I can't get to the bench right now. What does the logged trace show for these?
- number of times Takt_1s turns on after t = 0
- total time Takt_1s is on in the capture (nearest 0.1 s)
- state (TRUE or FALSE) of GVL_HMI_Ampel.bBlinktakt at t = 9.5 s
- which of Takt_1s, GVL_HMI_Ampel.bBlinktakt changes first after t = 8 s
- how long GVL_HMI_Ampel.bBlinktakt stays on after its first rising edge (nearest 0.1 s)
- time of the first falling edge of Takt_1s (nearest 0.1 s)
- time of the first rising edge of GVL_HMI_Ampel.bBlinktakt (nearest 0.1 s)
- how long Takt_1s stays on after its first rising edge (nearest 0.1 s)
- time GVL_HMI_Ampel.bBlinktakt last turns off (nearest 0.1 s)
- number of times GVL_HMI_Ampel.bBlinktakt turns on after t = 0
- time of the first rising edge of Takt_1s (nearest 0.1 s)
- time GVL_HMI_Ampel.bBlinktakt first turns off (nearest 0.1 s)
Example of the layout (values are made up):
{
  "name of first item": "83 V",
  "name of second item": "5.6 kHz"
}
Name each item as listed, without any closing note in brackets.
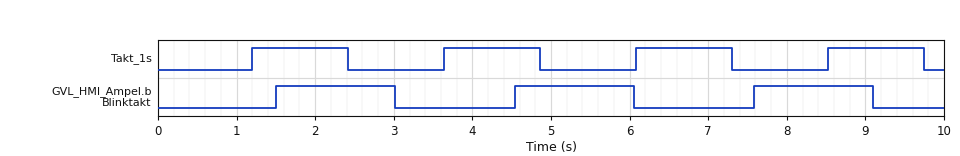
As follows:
{
  "number of times Takt_1s turns on after t = 0": "4",
  "total time Takt_1s is on in the capture": "4.9 s",
  "state (TRUE or FALSE) of GVL_HMI_Ampel.bBlinktakt at t = 9.5 s": "FALSE",
  "which of Takt_1s, GVL_HMI_Ampel.bBlinktakt changes first after t = 8 s": "Takt_1s",
  "how long GVL_HMI_Ampel.bBlinktakt stays on after its first rising edge": "1.5 s",
  "time of the first falling edge of Takt_1s": "2.4 s",
  "time of the first rising edge of GVL_HMI_Ampel.bBlinktakt": "1.5 s",
  "how long Takt_1s stays on after its first rising edge": "1.2 s",
  "time GVL_HMI_Ampel.bBlinktakt last turns off": "9.1 s",
  "number of times GVL_HMI_Ampel.bBlinktakt turns on after t = 0": "3",
  "time of the first rising edge of Takt_1s": "1.2 s",
  "time GVL_HMI_Ampel.bBlinktakt first turns off": "3.0 s"
}
